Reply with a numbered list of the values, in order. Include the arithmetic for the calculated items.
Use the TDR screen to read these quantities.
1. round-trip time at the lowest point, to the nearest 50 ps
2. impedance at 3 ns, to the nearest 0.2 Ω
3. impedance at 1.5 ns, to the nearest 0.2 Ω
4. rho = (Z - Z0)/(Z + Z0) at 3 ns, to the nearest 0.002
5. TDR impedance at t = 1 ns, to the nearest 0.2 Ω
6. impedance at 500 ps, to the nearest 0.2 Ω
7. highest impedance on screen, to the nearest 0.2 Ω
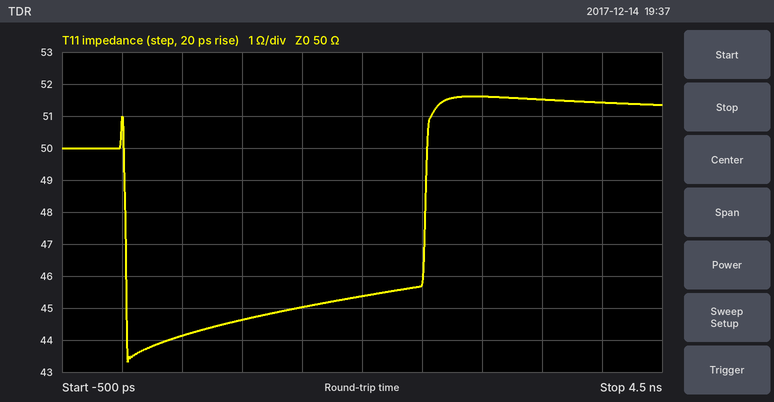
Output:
1. 50 ps
2. 51.6 Ω
3. 45.0 Ω
4. (51.6 − 50)/(51.6 + 50) ≈ +0.016
5. 44.6 Ω
6. 44.2 Ω
7. 51.6 Ω
